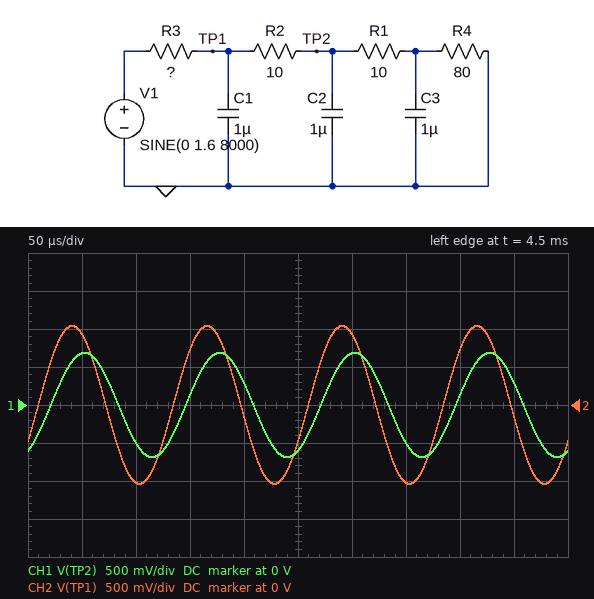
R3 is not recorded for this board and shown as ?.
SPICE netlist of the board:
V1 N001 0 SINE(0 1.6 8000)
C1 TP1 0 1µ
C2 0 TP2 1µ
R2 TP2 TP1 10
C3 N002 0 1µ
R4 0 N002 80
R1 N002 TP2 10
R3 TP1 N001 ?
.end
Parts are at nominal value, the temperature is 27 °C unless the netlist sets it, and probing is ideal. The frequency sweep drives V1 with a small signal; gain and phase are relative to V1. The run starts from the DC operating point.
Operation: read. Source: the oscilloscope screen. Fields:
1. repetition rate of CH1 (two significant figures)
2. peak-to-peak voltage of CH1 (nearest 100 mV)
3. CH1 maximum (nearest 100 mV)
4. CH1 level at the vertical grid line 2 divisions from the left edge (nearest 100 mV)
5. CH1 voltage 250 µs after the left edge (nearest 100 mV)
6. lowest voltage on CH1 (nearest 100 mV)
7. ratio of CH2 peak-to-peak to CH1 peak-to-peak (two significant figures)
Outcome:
8.0 kHz
1.4 V
700 mV
-500 mV
-600 mV
-700 mV
1.5
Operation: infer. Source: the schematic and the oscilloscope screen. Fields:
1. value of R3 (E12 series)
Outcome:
8.2 Ω
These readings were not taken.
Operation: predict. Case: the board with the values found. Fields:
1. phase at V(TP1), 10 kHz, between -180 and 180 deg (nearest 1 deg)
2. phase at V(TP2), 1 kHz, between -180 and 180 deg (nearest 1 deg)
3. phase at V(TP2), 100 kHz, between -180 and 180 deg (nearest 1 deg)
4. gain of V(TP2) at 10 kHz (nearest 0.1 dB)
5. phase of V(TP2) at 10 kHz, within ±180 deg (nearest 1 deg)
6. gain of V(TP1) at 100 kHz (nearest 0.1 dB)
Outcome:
-30 deg
-12 deg
-144 deg
-8.7 dB
-67 deg
-14.9 dB
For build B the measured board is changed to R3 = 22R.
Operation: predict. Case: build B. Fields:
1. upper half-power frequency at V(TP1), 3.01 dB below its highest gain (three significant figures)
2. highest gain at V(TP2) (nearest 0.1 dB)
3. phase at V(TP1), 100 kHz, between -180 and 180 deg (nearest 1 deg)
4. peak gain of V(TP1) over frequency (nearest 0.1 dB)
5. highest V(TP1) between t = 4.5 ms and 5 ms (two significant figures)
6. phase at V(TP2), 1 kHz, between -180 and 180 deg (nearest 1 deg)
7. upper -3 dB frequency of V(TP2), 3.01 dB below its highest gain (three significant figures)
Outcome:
3.11 kHz
-2.6 dB
-78 deg
-1.7 dB
580 mV
-21 deg
2.74 kHz
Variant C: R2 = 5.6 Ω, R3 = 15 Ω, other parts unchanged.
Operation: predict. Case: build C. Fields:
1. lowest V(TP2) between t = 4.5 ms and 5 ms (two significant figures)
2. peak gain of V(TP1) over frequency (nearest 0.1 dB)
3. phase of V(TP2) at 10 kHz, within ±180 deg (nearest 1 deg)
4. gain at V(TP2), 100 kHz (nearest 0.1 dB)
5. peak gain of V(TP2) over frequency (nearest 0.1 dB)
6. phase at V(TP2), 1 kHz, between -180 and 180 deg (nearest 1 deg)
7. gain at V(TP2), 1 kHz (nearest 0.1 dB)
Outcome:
-560 mV
-1.3 dB
-70 deg
-32.4 dB
-1.8 dB
-15 deg
-2.1 dB
